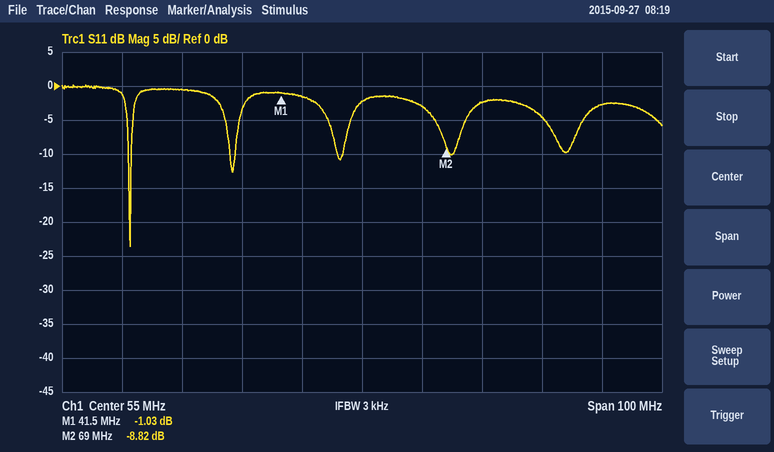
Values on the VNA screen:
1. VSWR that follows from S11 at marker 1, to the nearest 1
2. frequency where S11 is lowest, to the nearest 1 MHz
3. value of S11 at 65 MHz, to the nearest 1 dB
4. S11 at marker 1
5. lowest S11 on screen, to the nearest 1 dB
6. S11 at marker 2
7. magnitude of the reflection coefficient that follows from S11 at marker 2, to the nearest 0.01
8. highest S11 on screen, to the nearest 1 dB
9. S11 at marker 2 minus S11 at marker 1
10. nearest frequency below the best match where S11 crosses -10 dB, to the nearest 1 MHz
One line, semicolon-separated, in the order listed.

17; 16 MHz; -3 dB; -1.03 dB; -24 dB; -8.82 dB; 0.36; 0 dB; -7.79 dB; 16 MHz
